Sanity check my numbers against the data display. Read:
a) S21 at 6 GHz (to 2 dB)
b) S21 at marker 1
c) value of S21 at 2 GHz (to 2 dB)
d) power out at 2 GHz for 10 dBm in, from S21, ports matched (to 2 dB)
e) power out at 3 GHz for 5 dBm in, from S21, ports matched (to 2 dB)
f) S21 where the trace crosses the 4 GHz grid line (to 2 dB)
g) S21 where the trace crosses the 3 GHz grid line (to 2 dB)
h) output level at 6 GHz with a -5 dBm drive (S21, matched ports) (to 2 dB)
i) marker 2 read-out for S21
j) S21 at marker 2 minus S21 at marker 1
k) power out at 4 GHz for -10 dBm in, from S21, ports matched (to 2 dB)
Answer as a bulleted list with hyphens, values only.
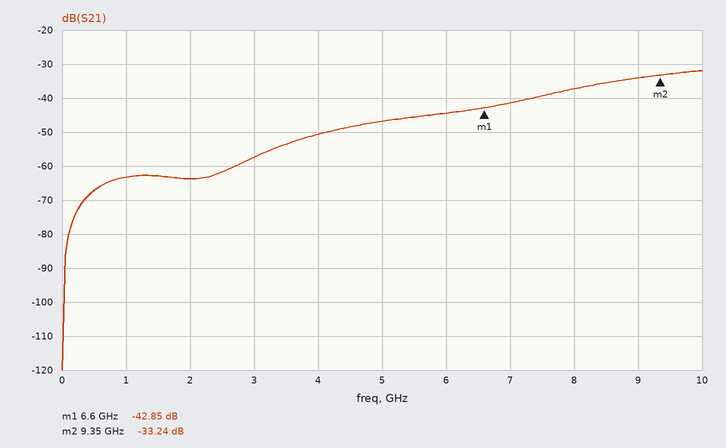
- -44 dB
- -42.85 dB
- -64 dB
- -54 dBm
- -52 dBm
- -50 dB
- -58 dB
- -50 dBm
- -33.24 dB
- 9.61 dB
- -60 dBm
